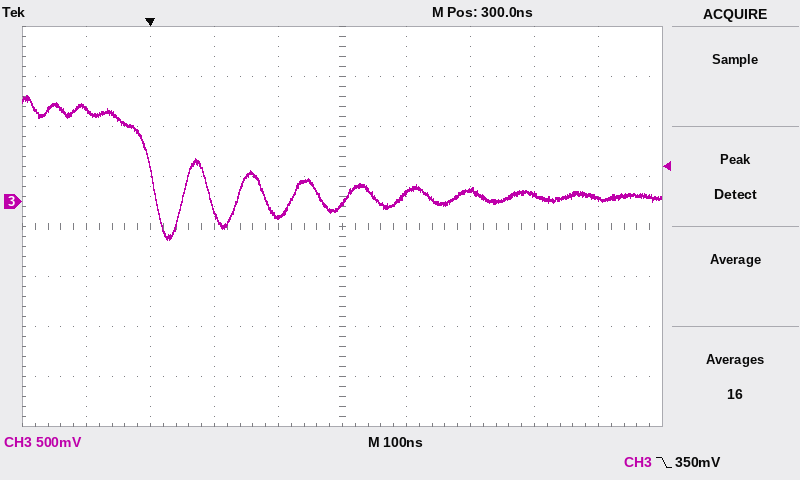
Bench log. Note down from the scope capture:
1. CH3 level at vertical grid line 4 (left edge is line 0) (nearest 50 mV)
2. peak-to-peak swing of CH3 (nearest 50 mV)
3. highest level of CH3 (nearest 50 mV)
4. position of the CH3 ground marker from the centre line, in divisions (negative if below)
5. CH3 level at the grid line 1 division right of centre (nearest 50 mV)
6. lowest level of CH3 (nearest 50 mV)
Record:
-150 mV
1.45 V
1.05 V
+0.5 div
100 mV
-400 mV
